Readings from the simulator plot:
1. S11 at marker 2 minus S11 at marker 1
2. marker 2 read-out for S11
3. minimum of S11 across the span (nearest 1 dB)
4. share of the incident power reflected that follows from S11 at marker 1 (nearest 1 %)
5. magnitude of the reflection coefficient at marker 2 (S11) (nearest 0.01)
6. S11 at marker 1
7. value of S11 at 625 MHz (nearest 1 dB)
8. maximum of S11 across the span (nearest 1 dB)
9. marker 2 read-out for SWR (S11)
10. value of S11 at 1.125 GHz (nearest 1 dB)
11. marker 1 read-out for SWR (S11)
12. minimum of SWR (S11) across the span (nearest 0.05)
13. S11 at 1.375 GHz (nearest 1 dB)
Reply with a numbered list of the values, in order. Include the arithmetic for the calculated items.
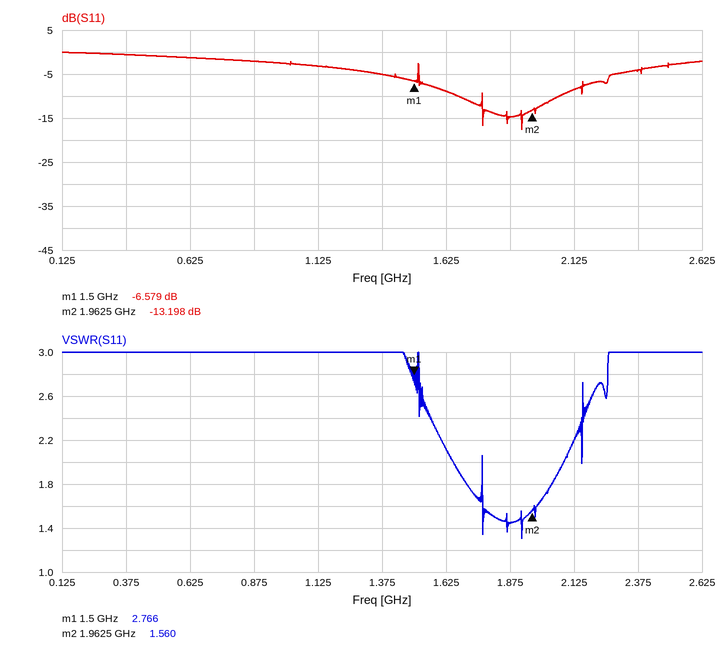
1. -13.198 − (-6.579) = -6.619 dB
2. -13.198 dB
3. -18 dB
4. 10^(-6.579/10) ≈ 22 %
5. 10^(-13.198/20) ≈ 0.22
6. -6.579 dB
7. -1 dB
8. 0 dB
9. 1.560
10. -3 dB
11. 2.766
12. 1.30
13. -5 dB
